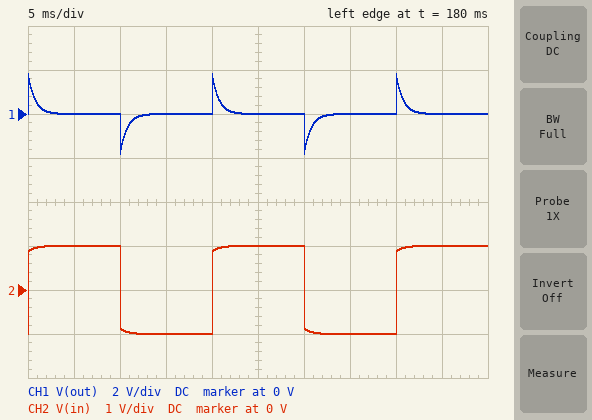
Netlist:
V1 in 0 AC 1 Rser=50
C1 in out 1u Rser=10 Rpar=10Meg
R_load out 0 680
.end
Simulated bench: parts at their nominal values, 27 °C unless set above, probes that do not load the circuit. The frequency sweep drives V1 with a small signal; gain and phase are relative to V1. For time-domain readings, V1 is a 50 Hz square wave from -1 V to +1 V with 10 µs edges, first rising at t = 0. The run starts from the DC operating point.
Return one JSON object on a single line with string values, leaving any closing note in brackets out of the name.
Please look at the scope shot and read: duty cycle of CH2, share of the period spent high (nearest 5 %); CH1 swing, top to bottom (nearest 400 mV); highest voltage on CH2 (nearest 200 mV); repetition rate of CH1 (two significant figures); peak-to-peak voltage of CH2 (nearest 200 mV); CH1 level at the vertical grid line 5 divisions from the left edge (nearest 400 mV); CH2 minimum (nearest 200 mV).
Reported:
{"duty cycle of CH2, share of the period spent high": "50 %", "CH1 swing, top to bottom": "3.6 V", "highest voltage on CH2": "1.0 V", "repetition rate of CH1": "50 Hz", "peak-to-peak voltage of CH2": "2.0 V", "CH1 level at the vertical grid line 5 divisions from the left edge": "0 V", "CH2 minimum": "-1.0 V"}
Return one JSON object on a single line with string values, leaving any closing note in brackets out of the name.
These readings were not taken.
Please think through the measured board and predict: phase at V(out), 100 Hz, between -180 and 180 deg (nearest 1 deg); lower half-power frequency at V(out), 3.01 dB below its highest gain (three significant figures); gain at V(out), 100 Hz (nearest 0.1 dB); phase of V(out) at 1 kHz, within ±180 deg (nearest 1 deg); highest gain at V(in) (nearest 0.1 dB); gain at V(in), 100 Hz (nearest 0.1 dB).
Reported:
{"phase at V(out), 100 Hz, between -180 and 180 deg": "65 deg", "lower half-power frequency at V(out), 3.01 dB below its highest gain": "215 Hz", "gain at V(out), 100 Hz": "-8.2 dB", "phase of V(out) at 1 kHz, within ±180 deg": "12 deg", "highest gain at V(in)": "0 dB", "gain at V(in), 100 Hz": "-0.1 dB"}
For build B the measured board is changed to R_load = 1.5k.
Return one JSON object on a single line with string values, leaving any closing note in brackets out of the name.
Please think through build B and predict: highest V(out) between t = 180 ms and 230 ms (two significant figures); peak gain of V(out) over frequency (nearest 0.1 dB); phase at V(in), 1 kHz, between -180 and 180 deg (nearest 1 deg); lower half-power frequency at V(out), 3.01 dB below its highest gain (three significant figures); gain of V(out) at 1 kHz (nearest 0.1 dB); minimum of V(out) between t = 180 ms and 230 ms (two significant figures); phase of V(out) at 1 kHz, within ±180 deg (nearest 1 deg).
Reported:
{"highest V(out) between t = 180 ms and 230 ms": "1.9 V", "peak gain of V(out) over frequency": "-0.3 dB", "phase at V(in), 1 kHz, between -180 and 180 deg": "0 deg", "lower half-power frequency at V(out), 3.01 dB below its highest gain": "102 Hz", "gain of V(out) at 1 kHz": "-0.4 dB", "minimum of V(out) between t = 180 ms and 230 ms": "-1.9 V", "phase of V(out) at 1 kHz, within ±180 deg": "6 deg"}
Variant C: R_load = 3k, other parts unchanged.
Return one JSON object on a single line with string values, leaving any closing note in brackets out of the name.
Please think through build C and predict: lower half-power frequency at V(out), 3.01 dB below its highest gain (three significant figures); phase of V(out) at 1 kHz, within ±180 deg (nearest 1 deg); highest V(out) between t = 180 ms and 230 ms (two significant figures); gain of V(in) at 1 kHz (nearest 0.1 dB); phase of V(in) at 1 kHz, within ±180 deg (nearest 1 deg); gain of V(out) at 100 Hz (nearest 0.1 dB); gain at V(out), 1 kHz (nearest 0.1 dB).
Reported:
{"lower half-power frequency at V(out), 3.01 dB below its highest gain": "52.0 Hz", "phase of V(out) at 1 kHz, within ±180 deg": "3 deg", "highest V(out) between t = 180 ms and 230 ms": "1.9 V", "gain of V(in) at 1 kHz": "-0.1 dB", "phase of V(in) at 1 kHz, within ±180 deg": "0 deg", "gain of V(out) at 100 Hz": "-1.2 dB", "gain at V(out), 1 kHz": "-0.2 dB"}
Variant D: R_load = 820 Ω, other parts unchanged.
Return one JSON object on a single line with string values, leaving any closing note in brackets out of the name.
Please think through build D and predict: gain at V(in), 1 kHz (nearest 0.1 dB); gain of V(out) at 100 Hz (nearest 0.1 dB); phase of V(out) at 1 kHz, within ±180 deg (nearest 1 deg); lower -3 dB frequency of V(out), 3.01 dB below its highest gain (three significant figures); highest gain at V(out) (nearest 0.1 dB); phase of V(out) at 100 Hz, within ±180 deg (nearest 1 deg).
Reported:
{"gain at V(in), 1 kHz": "-0.5 dB", "gain of V(out) at 100 Hz": "-6.9 dB", "phase of V(out) at 1 kHz, within ±180 deg": "10 deg", "lower -3 dB frequency of V(out), 3.01 dB below its highest gain": "181 Hz", "highest gain at V(out)": "-0.6 dB", "phase of V(out) at 100 Hz, within ±180 deg": "61 deg"}
